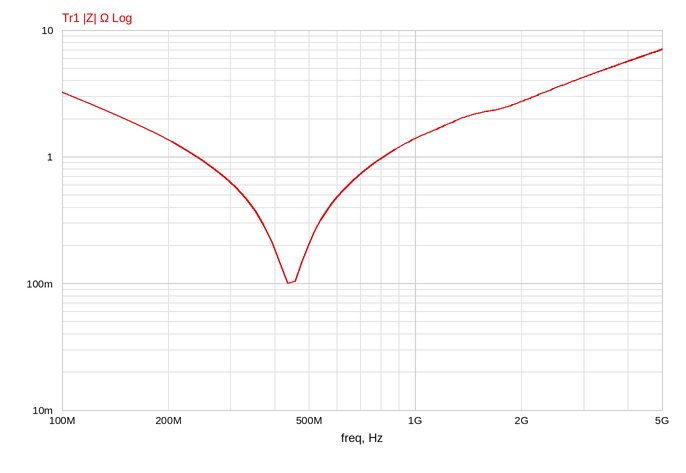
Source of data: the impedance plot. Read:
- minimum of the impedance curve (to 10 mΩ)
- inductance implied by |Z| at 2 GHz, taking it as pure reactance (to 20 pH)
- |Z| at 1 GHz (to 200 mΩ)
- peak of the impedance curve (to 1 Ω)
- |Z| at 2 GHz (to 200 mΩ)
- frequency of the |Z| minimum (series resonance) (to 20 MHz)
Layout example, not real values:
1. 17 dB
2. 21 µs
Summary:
1. 100 mΩ
2. 220 pH
3. 1.4 Ω
4. 7 Ω
5. 2.8 Ω
6. 440 MHz
